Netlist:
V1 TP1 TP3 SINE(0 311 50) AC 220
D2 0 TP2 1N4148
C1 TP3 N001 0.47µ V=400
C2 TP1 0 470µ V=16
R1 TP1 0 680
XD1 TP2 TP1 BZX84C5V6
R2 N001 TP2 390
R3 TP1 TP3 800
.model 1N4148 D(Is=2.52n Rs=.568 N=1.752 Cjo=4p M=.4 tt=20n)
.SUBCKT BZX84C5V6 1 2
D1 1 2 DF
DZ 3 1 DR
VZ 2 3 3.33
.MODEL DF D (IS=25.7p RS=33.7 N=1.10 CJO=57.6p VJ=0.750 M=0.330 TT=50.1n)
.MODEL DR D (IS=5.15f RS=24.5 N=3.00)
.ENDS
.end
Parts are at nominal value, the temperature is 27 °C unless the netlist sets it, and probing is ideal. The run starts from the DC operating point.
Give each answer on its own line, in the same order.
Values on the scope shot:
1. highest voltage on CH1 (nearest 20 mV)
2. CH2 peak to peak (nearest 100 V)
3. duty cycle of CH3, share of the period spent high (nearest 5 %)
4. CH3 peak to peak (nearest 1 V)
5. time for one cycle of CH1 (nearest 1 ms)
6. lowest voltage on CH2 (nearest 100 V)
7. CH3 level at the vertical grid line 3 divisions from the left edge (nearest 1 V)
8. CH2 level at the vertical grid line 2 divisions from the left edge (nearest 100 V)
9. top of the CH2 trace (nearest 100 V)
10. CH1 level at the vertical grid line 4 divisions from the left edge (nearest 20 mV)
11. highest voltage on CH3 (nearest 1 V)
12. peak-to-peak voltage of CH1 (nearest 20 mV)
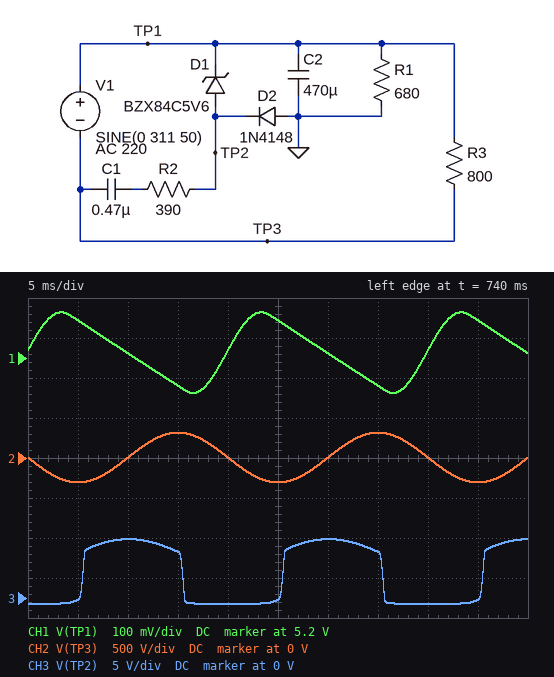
5.32 V
600 V
50 %
8 V
20 ms
-300 V
6 V
0 V
300 V
5.22 V
7 V
200 mV
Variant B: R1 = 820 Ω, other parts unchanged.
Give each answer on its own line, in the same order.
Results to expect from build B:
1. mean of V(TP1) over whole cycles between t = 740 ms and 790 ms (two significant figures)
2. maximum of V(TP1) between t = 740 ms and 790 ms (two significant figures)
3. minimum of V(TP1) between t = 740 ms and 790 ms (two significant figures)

5.3 V
5.4 V
5.2 V
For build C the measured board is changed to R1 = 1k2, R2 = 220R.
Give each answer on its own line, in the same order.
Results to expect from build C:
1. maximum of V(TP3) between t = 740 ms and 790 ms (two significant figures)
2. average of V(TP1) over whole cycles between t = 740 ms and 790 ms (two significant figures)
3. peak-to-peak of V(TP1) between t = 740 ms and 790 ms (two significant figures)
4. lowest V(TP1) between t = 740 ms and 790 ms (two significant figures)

320 V
5.5 V
130 mV
5.4 V
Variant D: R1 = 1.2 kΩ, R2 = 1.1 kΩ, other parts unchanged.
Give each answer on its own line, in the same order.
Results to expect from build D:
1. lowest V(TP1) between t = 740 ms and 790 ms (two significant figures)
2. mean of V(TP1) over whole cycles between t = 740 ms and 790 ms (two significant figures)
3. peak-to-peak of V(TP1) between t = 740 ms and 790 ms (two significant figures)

5.4 V
5.5 V
130 mV
